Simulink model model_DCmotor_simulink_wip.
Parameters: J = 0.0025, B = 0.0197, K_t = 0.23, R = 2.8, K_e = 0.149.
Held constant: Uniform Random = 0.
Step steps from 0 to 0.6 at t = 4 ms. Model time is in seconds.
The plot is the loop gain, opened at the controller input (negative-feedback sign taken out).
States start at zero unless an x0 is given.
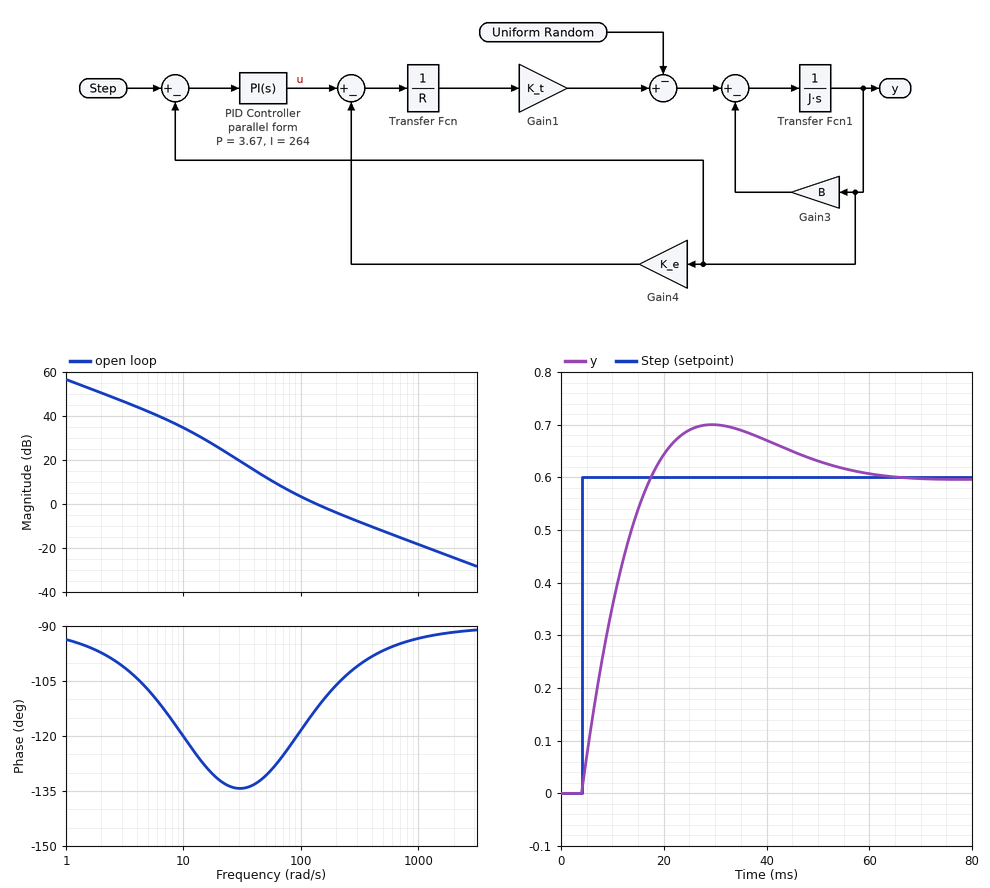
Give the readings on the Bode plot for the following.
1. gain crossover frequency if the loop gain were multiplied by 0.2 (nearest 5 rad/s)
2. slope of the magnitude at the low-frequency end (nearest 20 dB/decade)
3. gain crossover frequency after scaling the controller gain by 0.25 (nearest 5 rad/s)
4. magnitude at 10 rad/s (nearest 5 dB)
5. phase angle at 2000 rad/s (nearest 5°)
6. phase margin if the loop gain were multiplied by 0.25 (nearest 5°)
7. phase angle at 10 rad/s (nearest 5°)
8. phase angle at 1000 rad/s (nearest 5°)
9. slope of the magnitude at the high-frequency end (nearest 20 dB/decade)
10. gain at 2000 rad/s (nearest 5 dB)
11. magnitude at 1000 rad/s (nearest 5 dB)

45 rad/s
-20 dB/decade
50 rad/s
35 dB
-90°
50°
-120°
-95°
-20 dB/decade
-25 dB
-20 dB
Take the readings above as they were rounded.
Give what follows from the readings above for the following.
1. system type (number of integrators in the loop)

1
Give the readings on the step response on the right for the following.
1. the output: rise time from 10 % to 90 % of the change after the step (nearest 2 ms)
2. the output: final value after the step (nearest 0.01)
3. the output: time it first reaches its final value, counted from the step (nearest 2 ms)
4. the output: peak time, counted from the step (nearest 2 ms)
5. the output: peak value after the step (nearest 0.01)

10 ms
0.60
14 ms
26 ms
0.70
